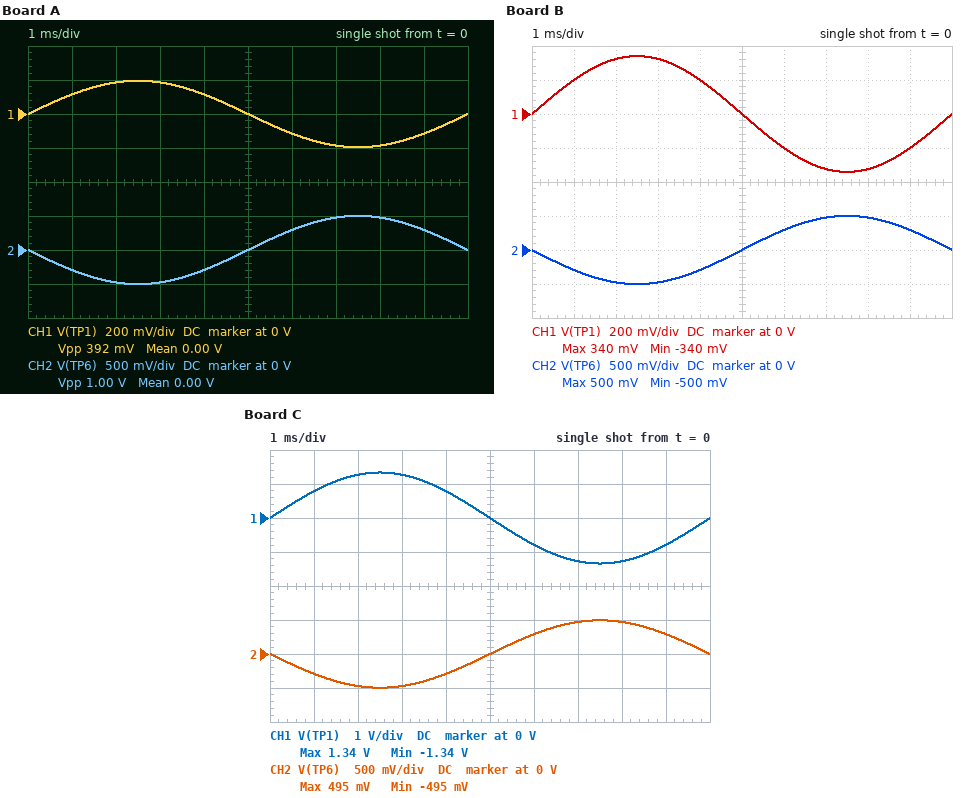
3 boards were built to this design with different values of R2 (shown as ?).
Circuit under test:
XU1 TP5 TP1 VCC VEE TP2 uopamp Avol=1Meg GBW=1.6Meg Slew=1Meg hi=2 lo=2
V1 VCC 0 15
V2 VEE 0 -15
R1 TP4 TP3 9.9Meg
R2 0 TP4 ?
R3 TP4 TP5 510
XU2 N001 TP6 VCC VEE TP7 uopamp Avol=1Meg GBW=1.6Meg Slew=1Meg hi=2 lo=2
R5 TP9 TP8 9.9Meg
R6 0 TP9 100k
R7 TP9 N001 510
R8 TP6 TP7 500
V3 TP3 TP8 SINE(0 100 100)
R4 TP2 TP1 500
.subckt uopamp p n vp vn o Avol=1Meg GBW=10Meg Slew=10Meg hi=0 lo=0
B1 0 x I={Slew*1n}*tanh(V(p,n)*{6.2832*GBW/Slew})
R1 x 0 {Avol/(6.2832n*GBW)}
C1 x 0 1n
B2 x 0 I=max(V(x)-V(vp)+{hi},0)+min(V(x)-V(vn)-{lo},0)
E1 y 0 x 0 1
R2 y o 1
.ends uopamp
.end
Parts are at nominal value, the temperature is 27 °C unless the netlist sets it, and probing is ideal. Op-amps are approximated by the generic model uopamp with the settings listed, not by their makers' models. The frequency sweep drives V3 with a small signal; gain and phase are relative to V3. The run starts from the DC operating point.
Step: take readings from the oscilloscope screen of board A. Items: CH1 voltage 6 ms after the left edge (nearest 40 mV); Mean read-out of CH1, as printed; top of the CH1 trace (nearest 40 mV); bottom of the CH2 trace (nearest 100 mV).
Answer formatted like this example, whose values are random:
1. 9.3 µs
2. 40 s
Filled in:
1. -120 mV
2. 0.00 V
3. 200 mV
4. -500 mV
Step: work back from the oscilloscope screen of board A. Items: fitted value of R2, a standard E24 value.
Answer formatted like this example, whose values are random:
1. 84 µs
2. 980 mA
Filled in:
1. 39 kΩ
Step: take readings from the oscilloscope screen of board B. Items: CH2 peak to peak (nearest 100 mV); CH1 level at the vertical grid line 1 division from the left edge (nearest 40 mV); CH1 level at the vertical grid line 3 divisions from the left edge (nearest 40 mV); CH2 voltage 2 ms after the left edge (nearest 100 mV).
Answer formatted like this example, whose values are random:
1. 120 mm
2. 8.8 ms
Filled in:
1. 1.0 V
2. 200 mV
3. 320 mV
4. -500 mV
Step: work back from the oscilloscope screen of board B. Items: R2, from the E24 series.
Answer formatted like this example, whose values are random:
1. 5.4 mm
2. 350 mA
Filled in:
1. 68 kΩ
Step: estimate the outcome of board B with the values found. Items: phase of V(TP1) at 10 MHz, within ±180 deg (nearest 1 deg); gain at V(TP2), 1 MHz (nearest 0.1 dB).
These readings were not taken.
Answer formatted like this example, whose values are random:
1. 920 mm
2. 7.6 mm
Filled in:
1. -81 deg
2. -50.8 dB
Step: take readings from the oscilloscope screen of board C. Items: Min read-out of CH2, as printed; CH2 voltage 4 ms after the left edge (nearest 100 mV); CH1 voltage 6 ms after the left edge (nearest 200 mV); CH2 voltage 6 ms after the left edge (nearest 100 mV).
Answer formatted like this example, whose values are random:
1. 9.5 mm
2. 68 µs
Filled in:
1. -495 mV
2. -300 mV
3. -800 mV
4. 300 mV
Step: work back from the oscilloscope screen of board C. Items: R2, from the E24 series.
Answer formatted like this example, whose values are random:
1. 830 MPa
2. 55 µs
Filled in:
1. 270 kΩ
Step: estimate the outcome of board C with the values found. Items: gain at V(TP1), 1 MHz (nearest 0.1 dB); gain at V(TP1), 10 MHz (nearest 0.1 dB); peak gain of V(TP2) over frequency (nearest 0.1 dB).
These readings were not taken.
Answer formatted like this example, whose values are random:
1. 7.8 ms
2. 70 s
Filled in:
1. -38.9 dB
2. -53.5 dB
3. -37.5 dB
